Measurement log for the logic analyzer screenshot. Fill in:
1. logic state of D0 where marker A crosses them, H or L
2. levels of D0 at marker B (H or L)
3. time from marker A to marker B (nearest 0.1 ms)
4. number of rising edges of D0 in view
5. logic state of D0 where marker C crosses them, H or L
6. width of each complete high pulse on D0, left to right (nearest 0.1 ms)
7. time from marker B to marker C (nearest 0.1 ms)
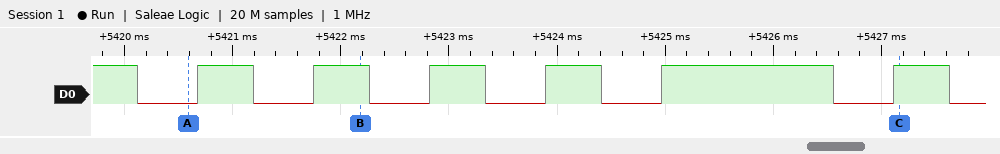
D0=L
D0=H
1.6 ms
6
D0=H
0.5 ms, 0.5 ms, 0.5 ms, 0.5 ms, 1.6 ms, 0.5 ms
5 ms
